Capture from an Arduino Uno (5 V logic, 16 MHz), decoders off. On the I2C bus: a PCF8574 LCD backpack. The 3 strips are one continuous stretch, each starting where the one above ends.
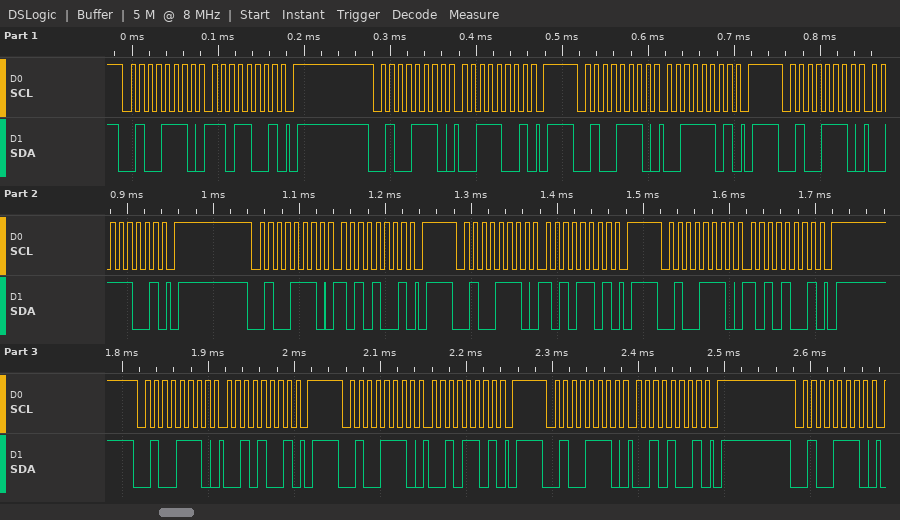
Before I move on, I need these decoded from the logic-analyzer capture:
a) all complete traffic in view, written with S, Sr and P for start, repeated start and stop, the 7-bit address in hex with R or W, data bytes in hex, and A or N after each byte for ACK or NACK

S 27W A D9 A P S 27W A 39 A P S 27W A 3D A P S 27W A 39 A P S 27W A A9 A P S 27W A AD A P S 27W A A9 A P S 27W A 29 A P S 27W A 2D A P S 27W A 29 A P S 27W A
